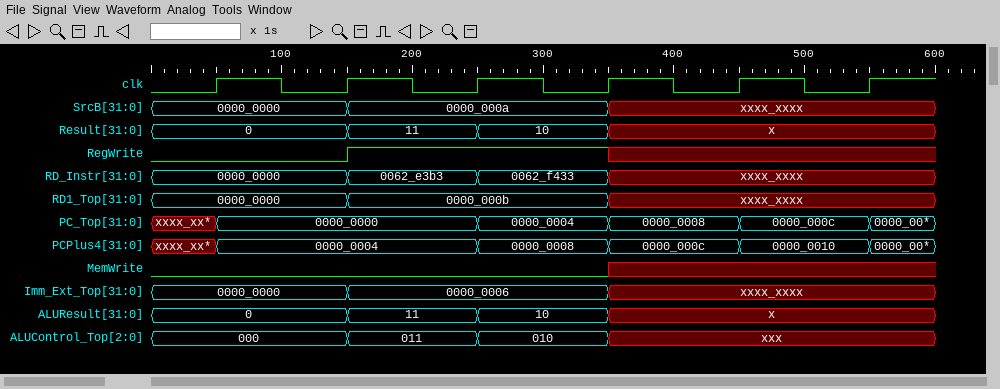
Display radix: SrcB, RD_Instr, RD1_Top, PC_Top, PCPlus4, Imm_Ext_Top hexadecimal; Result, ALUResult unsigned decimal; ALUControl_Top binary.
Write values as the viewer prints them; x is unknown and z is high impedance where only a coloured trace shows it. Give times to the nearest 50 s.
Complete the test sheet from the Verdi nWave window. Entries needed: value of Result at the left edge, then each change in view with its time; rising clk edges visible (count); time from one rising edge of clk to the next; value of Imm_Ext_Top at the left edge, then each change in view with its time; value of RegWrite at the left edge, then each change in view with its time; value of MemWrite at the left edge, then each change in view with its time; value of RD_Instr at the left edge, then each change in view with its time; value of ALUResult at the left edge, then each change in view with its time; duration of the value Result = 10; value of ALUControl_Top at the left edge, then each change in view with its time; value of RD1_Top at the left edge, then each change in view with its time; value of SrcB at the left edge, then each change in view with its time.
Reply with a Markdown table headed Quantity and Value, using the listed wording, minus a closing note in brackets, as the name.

| Quantity | Value |
|---|---|
| value of Result at the left edge, then each change in view with its time | 0, 11 at 150 s, 10 at 250 s, x at 350 s |
| rising clk edges visible | 6 |
| time from one rising edge of clk to the next | 100 s |
| value of Imm_Ext_Top at the left edge, then each change in view with its time | 0000_0000, 0000_0006 at 150 s, xxxx_xxxx at 350 s |
| value of RegWrite at the left edge, then each change in view with its time | 0, 1 at 150 s, x at 350 s |
| value of MemWrite at the left edge, then each change in view with its time | 0, x at 350 s |
| value of RD_Instr at the left edge, then each change in view with its time | 0000_0000, 0062_e3b3 at 150 s, 0062_f433 at 250 s, xxxx_xxxx at 350 s |
| value of ALUResult at the left edge, then each change in view with its time | 0, 11 at 150 s, 10 at 250 s, x at 350 s |
| duration of the value Result = 10 | 100 s |
| value of ALUControl_Top at the left edge, then each change in view with its time | 000, 011 at 150 s, 010 at 250 s, xxx at 350 s |
| value of RD1_Top at the left edge, then each change in view with its time | 0000_0000, 0000_000b at 150 s, xxxx_xxxx at 350 s |
| value of SrcB at the left edge, then each change in view with its time | 0000_0000, 0000_000a at 150 s, xxxx_xxxx at 350 s |
